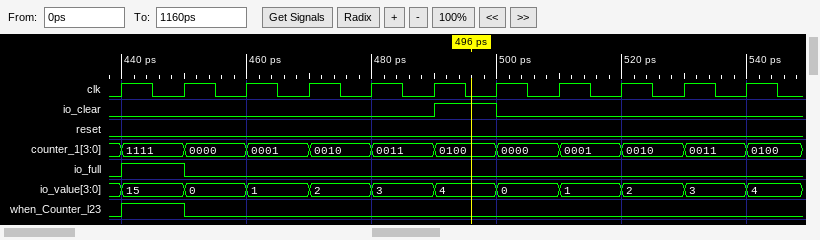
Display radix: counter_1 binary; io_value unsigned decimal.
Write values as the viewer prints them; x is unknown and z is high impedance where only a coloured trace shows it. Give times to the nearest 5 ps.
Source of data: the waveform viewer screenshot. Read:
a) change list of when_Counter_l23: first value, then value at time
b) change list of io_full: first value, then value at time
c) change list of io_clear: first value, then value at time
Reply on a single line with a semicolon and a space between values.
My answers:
0, 1 at 440 ps, 0 at 450 ps; 0, 1 at 440 ps, 0 at 450 ps; 0, 1 at 490 ps, 0 at 500 ps
